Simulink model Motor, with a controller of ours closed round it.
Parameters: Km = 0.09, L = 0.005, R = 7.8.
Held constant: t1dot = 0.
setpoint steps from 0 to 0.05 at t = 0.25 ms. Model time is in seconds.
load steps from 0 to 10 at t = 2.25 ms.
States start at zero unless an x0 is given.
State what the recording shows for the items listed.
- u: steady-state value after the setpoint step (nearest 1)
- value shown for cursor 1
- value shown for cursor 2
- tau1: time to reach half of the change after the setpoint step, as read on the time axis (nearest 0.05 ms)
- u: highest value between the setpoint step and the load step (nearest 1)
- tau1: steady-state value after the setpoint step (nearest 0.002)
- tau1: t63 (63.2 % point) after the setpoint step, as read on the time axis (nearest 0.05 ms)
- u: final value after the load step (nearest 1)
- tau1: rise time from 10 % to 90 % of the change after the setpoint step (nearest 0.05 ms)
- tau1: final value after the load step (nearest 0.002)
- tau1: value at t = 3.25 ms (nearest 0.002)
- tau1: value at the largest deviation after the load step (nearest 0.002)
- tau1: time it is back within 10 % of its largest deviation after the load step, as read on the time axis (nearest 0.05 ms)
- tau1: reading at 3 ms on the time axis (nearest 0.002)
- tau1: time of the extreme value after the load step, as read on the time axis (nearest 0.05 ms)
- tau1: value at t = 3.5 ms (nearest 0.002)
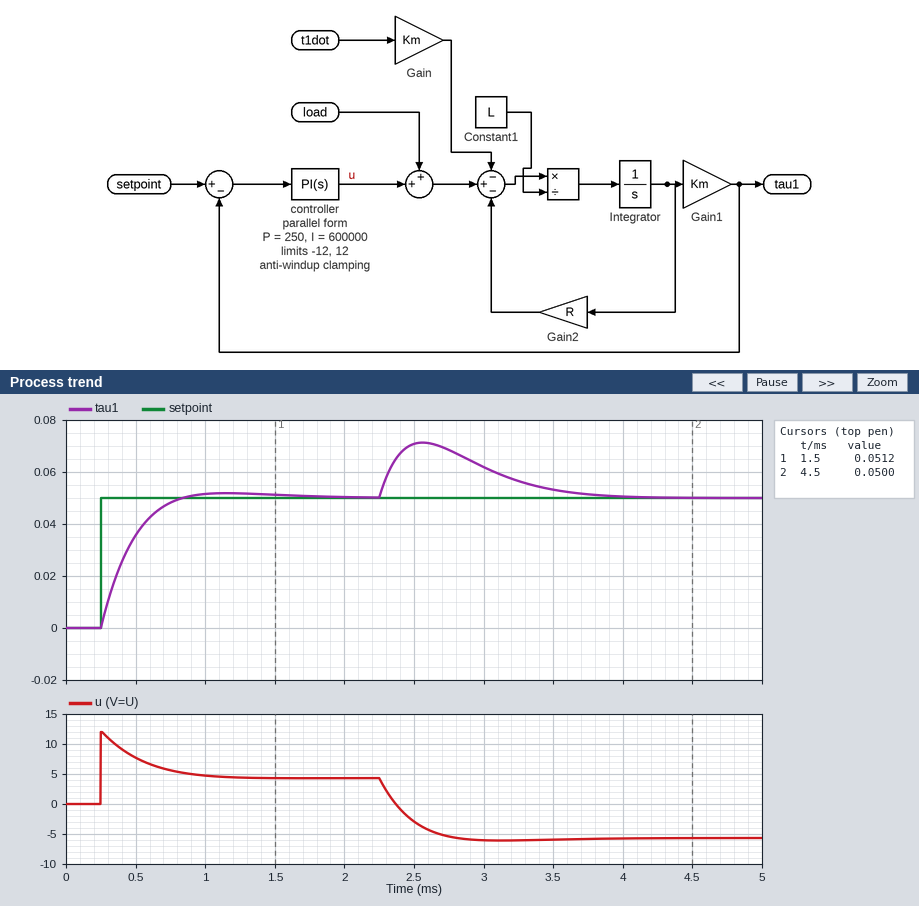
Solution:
4
0.0512
0.0500
0.40 ms
12
0.050
0.45 ms
-6
0.40 ms
0.050
0.056
0.072
3.65 ms
0.062
2.55 ms
0.054
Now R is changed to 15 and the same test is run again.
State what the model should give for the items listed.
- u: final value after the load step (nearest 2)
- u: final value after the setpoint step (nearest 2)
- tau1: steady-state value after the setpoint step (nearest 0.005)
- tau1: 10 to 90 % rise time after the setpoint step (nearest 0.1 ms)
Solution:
-2
8
0.050
0.7 ms
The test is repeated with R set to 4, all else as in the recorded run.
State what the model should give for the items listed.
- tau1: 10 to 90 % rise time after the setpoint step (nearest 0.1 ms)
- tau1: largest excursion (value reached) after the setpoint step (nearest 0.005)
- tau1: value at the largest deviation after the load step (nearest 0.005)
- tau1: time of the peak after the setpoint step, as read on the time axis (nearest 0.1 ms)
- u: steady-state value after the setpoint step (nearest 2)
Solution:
0.3 ms
0.055
0.075
1.0 ms
2
